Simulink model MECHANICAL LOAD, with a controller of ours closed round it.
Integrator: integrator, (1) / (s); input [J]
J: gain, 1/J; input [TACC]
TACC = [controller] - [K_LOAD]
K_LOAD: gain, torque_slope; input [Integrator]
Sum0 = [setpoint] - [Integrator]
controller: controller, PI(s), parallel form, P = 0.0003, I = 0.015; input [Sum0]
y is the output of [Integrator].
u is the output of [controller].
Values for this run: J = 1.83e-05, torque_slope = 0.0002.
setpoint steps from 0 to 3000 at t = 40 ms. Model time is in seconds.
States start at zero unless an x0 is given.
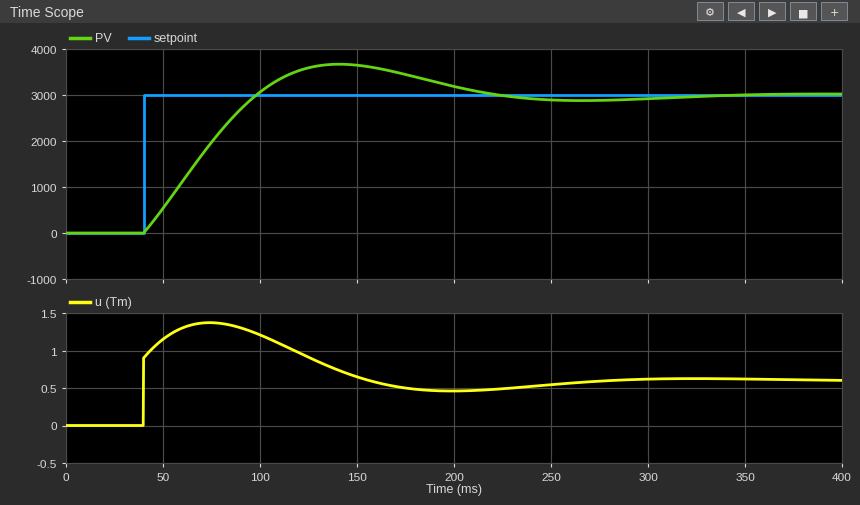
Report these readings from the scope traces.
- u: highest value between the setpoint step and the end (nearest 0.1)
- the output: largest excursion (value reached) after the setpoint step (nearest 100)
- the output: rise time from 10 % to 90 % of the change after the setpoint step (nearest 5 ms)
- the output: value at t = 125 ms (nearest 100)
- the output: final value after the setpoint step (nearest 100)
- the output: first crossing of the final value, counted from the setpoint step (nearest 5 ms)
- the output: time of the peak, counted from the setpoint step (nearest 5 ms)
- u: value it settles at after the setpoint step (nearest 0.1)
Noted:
1.4
3700
45 ms
3600
3000
60 ms
100 ms
0.6
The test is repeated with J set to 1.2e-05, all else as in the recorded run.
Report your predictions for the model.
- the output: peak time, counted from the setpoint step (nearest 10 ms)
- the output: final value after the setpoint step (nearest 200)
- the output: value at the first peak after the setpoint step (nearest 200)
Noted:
80 ms
3000
3400
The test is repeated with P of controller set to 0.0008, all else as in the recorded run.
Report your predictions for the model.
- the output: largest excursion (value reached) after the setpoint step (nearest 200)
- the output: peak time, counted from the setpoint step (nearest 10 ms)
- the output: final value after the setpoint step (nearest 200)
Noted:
3200
90 ms
3000
